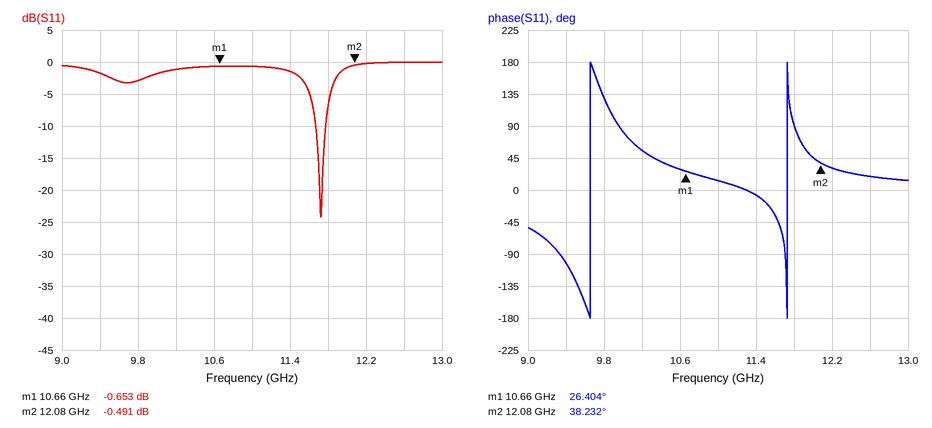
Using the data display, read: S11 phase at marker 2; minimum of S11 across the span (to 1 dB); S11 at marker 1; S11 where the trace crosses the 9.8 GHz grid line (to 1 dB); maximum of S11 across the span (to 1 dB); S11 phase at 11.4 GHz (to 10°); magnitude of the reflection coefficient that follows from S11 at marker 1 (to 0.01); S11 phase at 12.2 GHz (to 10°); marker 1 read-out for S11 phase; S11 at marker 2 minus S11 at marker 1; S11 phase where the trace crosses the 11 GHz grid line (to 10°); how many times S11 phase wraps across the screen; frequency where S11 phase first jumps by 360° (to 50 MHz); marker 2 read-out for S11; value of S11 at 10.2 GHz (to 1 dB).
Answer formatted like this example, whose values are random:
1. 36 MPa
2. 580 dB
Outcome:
1. 38.232°
2. -24 dB
3. -0.653 dB
4. -3 dB
5. 0 dB
6. -10°
7. 0.93
8. 30°
9. 26.404°
10. 0.162 dB
11. 10°
12. 2
13. 9.65 GHz
14. -0.491 dB
15. -1 dB
